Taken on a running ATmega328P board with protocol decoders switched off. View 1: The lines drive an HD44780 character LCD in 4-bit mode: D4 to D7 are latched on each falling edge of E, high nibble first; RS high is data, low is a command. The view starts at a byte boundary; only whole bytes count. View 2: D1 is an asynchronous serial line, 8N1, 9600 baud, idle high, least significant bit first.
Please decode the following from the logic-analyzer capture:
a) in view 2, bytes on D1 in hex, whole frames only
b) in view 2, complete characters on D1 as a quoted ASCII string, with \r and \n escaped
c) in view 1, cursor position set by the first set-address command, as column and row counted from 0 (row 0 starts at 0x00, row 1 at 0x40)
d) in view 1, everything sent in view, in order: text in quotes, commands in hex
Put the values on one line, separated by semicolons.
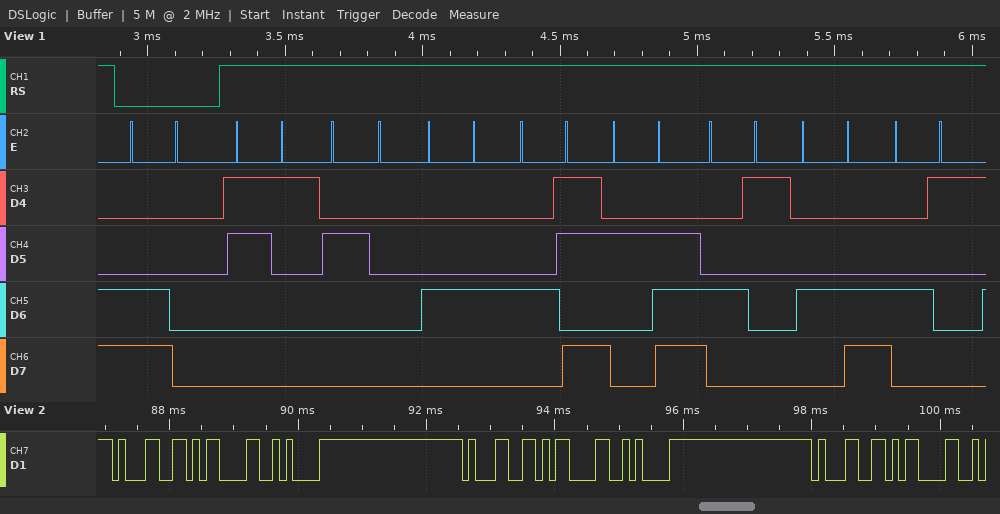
31 0D 0A 31 0D 0A 31 0D; "1\r\n1\r\n1\r"; column 0, row 1; 0xC0 "1 DK.ALA"
